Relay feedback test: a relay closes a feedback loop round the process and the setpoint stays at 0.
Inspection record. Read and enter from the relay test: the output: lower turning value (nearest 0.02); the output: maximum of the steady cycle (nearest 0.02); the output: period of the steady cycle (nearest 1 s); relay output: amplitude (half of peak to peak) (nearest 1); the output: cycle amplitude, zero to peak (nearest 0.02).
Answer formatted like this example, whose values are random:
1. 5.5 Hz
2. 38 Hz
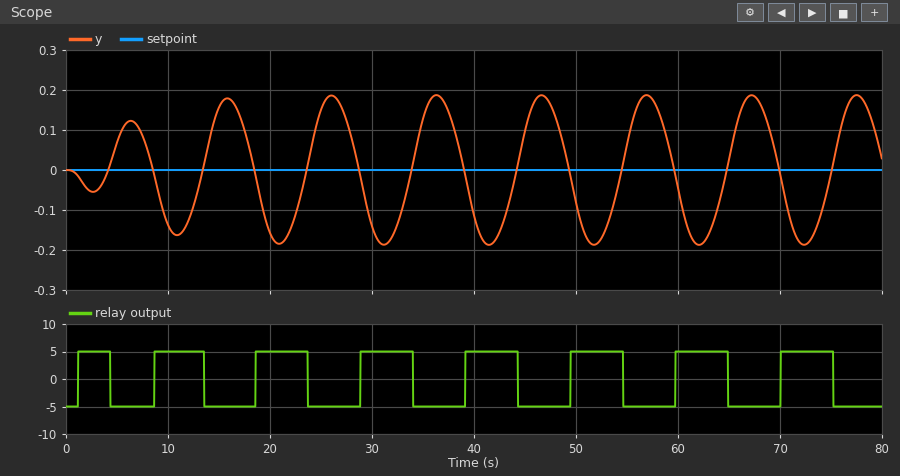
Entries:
1. -0.18
2. 0.18
3. 10 s
4. 5
5. 0.18
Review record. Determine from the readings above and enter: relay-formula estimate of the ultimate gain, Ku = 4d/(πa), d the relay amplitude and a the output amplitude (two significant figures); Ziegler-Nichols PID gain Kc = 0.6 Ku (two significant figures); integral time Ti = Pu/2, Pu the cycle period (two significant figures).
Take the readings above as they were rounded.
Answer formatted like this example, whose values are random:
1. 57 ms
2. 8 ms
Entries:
1. 35
2. 21
3. 5.0 s
